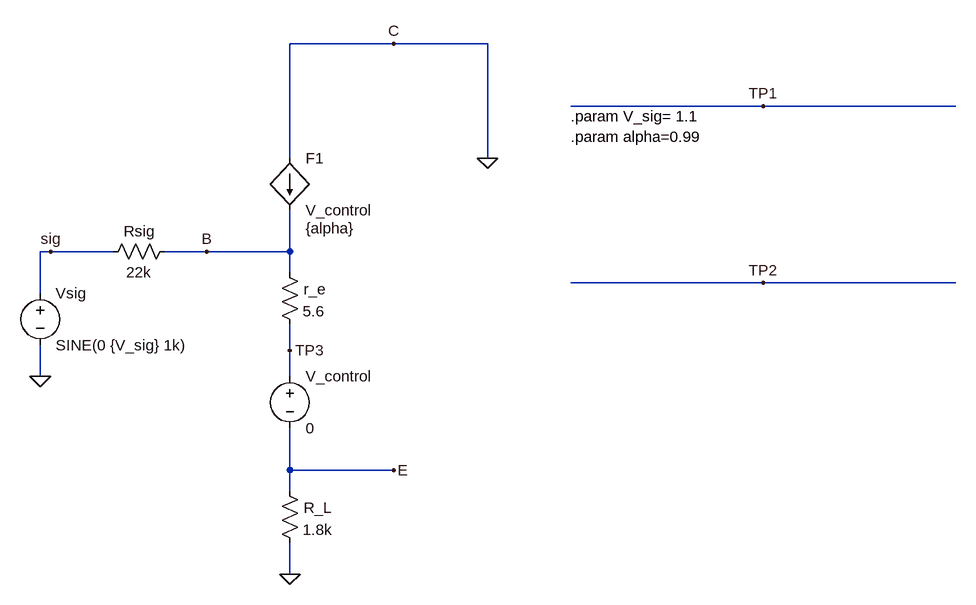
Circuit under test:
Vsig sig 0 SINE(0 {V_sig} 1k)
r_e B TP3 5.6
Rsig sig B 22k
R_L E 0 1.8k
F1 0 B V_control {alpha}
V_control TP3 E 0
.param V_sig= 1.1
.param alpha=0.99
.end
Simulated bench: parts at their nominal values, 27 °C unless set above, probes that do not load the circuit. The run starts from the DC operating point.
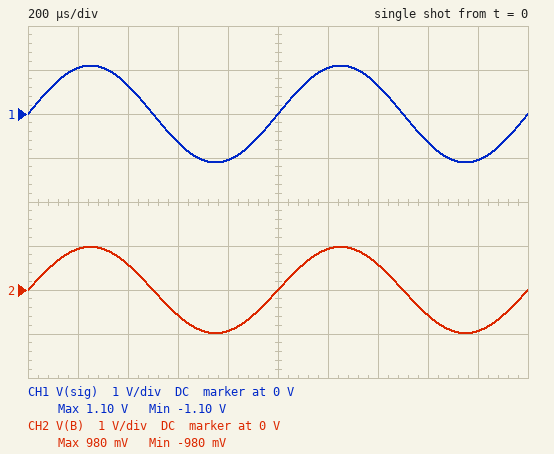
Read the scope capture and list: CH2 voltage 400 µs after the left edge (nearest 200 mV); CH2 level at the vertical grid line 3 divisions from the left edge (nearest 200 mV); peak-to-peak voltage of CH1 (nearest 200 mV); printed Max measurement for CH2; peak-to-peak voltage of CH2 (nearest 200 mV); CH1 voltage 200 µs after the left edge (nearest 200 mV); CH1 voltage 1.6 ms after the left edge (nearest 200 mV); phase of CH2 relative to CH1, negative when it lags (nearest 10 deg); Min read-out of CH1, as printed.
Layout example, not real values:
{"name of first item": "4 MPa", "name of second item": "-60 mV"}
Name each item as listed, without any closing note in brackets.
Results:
{"CH2 voltage 400 µs after the left edge": "600 mV", "CH2 level at the vertical grid line 3 divisions from the left edge": "-600 mV", "peak-to-peak voltage of CH1": "2.2 V", "printed Max measurement for CH2": "980 mV", "peak-to-peak voltage of CH2": "2.0 V", "CH1 voltage 200 µs after the left edge": "1.0 V", "CH1 voltage 1.6 ms after the left edge": "-600 mV", "phase of CH2 relative to CH1, negative when it lags": "0 deg", "Min read-out of CH1, as printed": "-1.10 V"}
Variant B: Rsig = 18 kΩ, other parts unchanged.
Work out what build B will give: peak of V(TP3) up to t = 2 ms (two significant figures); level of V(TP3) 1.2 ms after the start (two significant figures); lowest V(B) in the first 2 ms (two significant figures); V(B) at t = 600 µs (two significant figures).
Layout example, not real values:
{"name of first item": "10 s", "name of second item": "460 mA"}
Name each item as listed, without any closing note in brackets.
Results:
{"peak of V(TP3) up to t = 2 ms": "1.0 V", "level of V(TP3) 1.2 ms after the start": "950 mV", "lowest V(B) in the first 2 ms": "-1.0 V", "V(B) at t = 600 µs": "-590 mV"}
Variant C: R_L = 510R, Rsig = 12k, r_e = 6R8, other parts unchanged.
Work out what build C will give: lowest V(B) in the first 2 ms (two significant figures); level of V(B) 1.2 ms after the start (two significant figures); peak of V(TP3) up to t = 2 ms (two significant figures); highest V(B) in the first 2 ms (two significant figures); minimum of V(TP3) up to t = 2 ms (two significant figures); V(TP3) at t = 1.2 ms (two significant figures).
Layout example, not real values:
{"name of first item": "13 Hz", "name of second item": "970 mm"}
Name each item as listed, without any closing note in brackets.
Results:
{"lowest V(B) in the first 2 ms": "-890 mV", "level of V(B) 1.2 ms after the start": "850 mV", "peak of V(TP3) up to t = 2 ms": "880 mV", "highest V(B) in the first 2 ms": "890 mV", "minimum of V(TP3) up to t = 2 ms": "-880 mV", "V(TP3) at t = 1.2 ms": "840 mV"}
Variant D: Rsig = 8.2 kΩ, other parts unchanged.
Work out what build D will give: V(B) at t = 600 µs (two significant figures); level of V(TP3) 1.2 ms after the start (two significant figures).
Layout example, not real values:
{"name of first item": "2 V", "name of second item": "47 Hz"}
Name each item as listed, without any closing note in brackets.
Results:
{"V(B) at t = 600 µs": "-620 mV", "level of V(TP3) 1.2 ms after the start": "1.0 V"}
